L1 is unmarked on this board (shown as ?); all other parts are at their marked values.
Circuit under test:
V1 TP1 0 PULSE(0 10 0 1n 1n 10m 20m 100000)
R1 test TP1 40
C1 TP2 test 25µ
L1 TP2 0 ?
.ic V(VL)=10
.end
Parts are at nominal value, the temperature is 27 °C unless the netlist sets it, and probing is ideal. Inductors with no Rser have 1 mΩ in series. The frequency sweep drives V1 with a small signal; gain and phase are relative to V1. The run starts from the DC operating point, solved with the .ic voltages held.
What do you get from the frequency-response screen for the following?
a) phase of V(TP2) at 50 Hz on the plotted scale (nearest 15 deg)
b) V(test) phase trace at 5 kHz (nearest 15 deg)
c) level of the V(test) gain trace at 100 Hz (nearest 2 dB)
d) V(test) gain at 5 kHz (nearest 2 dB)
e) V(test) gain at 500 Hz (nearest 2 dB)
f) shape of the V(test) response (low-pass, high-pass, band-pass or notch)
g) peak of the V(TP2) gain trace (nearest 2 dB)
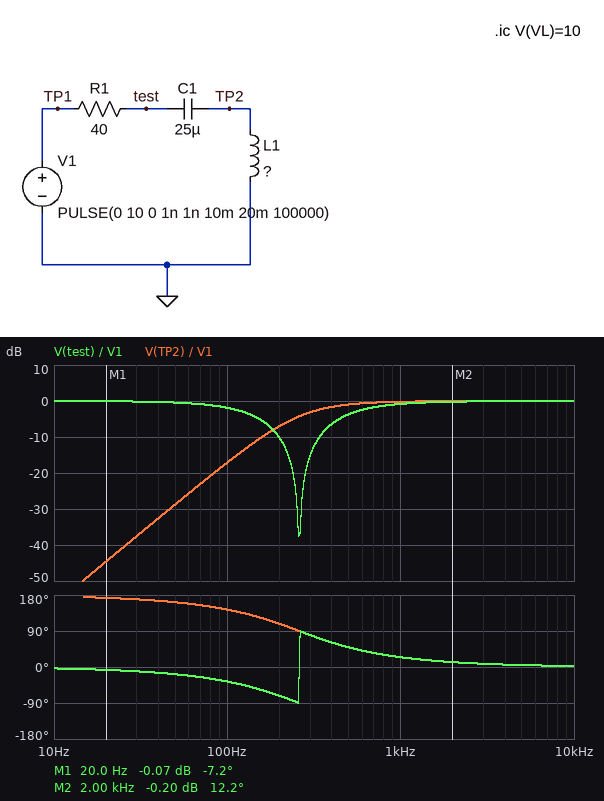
165 deg
0 deg
-2 dB
0 dB
-4 dB
notch
0 dB
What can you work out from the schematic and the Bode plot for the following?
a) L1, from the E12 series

15 mH
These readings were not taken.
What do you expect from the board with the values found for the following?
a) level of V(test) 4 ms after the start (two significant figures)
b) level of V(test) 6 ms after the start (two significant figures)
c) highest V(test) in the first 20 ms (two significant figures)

10 V
10 V
10 V
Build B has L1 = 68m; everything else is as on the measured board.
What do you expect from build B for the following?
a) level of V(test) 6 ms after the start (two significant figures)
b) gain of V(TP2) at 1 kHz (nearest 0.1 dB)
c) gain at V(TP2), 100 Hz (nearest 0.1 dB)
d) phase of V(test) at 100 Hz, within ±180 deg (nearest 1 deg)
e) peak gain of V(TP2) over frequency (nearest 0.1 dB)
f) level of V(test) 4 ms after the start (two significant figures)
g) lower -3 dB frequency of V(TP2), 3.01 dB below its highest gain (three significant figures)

11 V
0.1 dB
-0.5 dB
-62 deg
3.0 dB
9.2 V
103 Hz
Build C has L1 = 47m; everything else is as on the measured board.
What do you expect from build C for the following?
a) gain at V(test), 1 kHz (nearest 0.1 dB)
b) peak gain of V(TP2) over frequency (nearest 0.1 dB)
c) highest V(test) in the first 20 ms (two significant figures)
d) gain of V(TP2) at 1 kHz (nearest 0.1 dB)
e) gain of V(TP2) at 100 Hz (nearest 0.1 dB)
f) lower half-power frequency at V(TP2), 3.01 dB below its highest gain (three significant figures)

-0.1 dB
1.7 dB
11 V
0.1 dB
-5.0 dB
124 Hz
